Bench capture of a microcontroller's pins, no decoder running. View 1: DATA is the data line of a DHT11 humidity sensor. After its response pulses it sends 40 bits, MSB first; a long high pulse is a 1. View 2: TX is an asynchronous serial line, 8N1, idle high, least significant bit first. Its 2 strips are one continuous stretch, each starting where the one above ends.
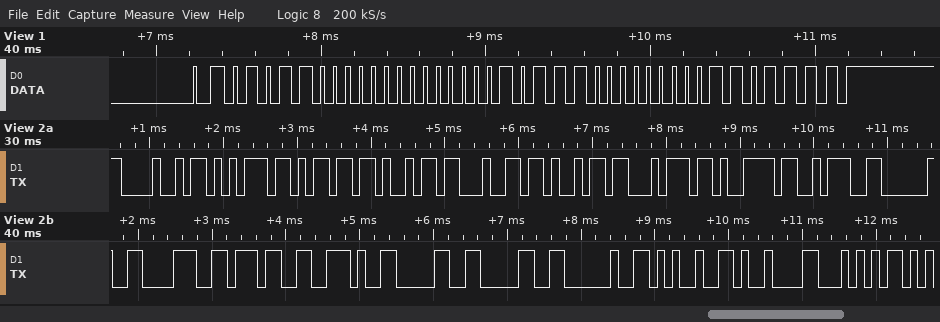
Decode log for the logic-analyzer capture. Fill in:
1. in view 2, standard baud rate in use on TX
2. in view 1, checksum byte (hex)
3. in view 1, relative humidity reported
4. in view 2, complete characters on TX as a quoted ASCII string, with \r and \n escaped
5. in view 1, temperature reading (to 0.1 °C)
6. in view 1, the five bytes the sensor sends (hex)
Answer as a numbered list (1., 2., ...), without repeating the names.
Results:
1. 9600 baud
2. 0x6F
3. 88 %
4. "Humidity: 87.00 %\tT"
5. 23.0 °C
6. 58 00 17 00 6F
